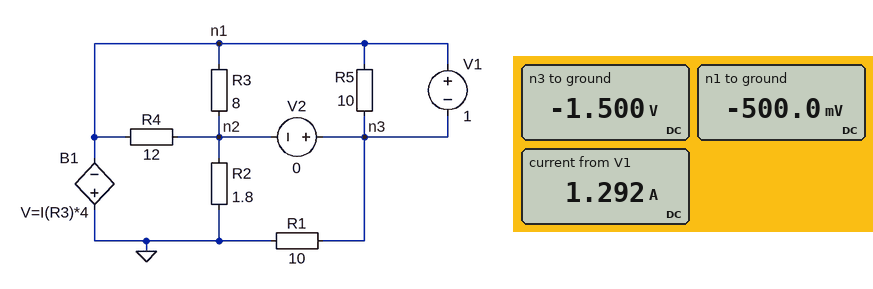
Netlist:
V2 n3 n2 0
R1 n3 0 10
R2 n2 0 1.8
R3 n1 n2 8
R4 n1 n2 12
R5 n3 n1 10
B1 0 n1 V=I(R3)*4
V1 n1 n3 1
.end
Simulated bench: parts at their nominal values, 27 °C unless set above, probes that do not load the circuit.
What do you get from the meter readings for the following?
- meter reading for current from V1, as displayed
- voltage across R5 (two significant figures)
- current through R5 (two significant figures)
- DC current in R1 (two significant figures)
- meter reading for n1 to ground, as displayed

1.292 A
1.0 V
100 mA
150 mA
-500.0 mV
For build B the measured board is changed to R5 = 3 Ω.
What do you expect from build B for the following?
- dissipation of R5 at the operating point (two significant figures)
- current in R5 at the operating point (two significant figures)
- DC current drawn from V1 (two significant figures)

330 mW
330 mA
1.5 A
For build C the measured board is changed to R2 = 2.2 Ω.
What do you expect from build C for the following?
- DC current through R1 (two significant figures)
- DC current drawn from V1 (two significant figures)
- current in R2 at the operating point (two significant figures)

150 mA
1.1 A
680 mA
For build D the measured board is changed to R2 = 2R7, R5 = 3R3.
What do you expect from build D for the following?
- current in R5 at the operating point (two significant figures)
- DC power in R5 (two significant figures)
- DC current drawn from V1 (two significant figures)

300 mA
300 mW
1.2 A
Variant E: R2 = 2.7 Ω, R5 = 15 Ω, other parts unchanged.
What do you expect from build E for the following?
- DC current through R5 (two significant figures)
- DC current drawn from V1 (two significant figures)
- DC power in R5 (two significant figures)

67 mA
980 mA
67 mW
